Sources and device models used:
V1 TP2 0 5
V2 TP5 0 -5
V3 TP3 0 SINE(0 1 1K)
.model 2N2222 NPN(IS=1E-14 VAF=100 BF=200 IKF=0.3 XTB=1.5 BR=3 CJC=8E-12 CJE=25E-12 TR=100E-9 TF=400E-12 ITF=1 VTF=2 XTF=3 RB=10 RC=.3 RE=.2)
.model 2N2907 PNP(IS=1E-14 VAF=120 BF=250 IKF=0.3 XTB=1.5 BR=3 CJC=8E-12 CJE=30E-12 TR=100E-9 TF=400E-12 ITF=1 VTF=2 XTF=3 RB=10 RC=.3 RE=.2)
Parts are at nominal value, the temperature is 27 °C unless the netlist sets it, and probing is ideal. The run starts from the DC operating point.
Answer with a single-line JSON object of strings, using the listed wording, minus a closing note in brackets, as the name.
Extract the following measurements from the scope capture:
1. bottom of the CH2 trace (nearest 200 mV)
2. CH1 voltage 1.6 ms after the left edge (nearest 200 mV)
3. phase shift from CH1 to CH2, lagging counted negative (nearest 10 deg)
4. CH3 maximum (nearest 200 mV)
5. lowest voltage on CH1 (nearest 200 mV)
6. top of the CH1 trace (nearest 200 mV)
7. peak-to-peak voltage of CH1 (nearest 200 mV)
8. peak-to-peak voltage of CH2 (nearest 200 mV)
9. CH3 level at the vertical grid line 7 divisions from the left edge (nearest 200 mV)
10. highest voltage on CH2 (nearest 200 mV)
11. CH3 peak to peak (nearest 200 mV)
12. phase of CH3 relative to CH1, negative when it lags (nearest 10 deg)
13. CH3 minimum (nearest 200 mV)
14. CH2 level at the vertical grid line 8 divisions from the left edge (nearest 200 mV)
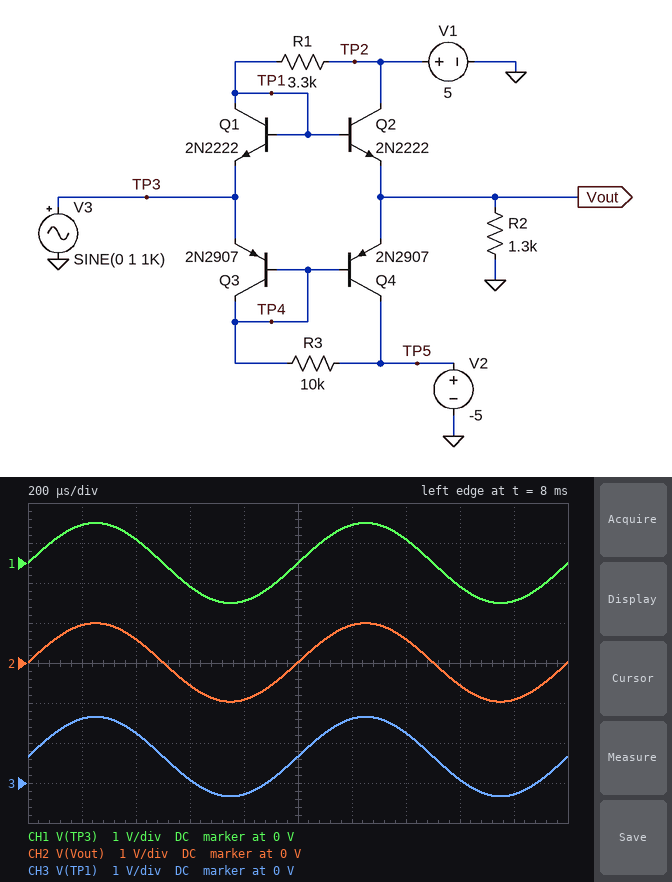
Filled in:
{"bottom of the CH2 trace": "-1.0 V", "CH1 voltage 1.6 ms after the left edge": "-600 mV", "phase shift from CH1 to CH2, lagging counted negative": "0 deg", "CH3 maximum": "1.6 V", "lowest voltage on CH1": "-1.0 V", "top of the CH1 trace": "1.0 V", "peak-to-peak voltage of CH1": "2.0 V", "peak-to-peak voltage of CH2": "2.0 V", "CH3 level at the vertical grid line 7 divisions from the left edge": "1.2 V", "highest voltage on CH2": "1.0 V", "CH3 peak to peak": "2.0 V", "phase of CH3 relative to CH1, negative when it lags": "0 deg", "CH3 minimum": "-400 mV", "CH2 level at the vertical grid line 8 divisions from the left edge": "-600 mV"}
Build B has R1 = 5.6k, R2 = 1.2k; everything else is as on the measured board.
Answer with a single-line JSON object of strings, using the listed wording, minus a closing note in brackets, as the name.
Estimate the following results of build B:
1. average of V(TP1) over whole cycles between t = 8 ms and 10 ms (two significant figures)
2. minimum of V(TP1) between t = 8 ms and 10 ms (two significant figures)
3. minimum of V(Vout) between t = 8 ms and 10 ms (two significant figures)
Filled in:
{"average of V(TP1) over whole cycles between t = 8 ms and 10 ms": "650 mV", "minimum of V(TP1) between t = 8 ms and 10 ms": "-350 mV", "minimum of V(Vout) between t = 8 ms and 10 ms": "-970 mV"}
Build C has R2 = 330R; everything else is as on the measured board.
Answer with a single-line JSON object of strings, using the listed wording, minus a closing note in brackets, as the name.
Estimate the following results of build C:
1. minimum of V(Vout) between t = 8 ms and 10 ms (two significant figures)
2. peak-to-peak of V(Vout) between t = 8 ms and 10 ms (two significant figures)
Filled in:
{"minimum of V(Vout) between t = 8 ms and 10 ms": "-940 mV", "peak-to-peak of V(Vout) between t = 8 ms and 10 ms": "1.9 V"}
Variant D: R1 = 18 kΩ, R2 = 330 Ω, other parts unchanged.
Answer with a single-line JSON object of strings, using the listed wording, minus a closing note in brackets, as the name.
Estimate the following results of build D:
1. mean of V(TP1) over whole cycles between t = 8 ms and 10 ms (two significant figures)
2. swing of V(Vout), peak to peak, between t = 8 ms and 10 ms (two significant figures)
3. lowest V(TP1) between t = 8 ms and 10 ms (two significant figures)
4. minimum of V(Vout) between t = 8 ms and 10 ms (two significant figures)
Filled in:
{"mean of V(TP1) over whole cycles between t = 8 ms and 10 ms": "620 mV", "swing of V(Vout), peak to peak, between t = 8 ms and 10 ms": "1.9 V", "lowest V(TP1) between t = 8 ms and 10 ms": "-380 mV", "minimum of V(Vout) between t = 8 ms and 10 ms": "-940 mV"}
